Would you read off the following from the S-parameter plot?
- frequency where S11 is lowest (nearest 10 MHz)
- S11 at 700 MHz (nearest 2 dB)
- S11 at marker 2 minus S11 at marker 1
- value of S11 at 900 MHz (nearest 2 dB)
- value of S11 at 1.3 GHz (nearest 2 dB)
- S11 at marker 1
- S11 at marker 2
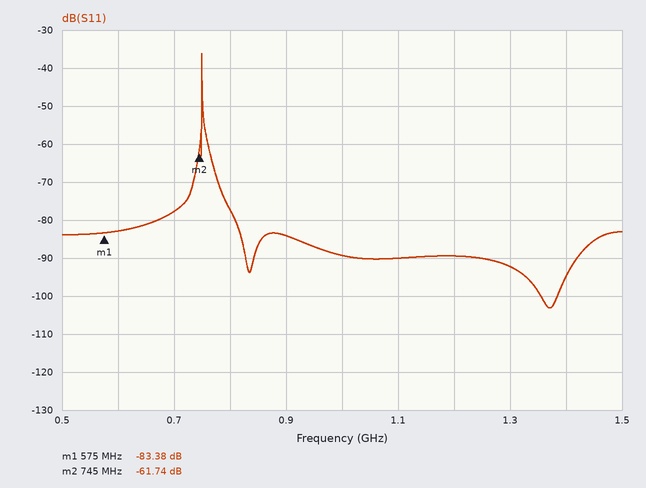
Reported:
1.37 GHz
-78 dB
21.64 dB
-84 dB
-92 dB
-83.38 dB
-61.74 dB
